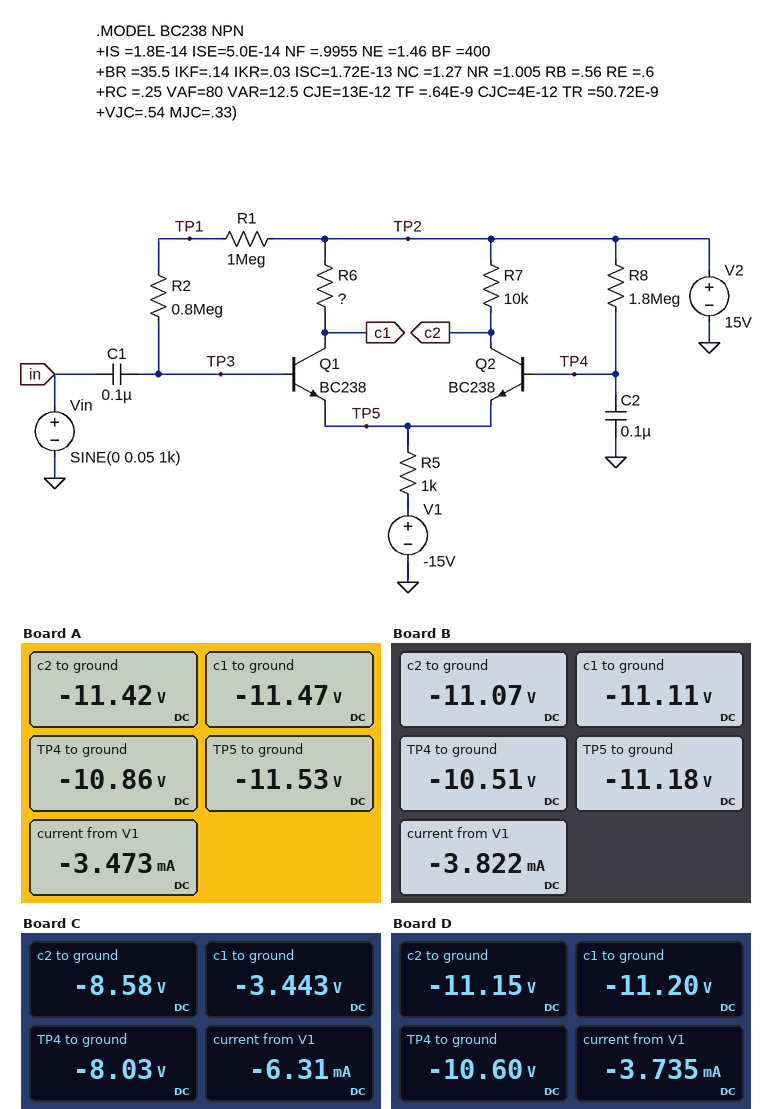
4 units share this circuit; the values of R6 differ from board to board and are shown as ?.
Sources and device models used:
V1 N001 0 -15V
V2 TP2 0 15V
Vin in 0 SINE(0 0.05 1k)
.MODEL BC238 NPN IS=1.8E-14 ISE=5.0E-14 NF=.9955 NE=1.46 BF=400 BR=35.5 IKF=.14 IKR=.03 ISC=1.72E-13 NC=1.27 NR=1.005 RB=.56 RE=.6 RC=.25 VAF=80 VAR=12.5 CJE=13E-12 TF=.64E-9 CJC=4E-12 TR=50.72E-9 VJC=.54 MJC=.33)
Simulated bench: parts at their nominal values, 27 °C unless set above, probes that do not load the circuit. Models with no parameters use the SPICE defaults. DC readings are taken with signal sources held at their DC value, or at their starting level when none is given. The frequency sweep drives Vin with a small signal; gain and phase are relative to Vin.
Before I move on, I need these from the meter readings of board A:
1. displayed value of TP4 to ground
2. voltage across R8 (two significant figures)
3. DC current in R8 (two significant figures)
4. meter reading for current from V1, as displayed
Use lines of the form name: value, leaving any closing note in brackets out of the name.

displayed value of TP4 to ground: -10.86 V
voltage across R8: 26 V
DC current in R8: 14 µA
meter reading for current from V1, as displayed: -3.473 mA
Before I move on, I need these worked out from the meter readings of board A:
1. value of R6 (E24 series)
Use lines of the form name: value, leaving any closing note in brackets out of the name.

value of R6: 33 kΩ
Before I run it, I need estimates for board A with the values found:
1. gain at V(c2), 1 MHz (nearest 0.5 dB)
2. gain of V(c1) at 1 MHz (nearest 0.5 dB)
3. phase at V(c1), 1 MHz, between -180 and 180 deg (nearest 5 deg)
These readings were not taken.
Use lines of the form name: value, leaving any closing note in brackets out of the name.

gain at V(c2), 1 MHz: 23.0 dB
gain of V(c1) at 1 MHz: 14.5 dB
phase at V(c1), 1 MHz, between -180 and 180 deg: 155 deg
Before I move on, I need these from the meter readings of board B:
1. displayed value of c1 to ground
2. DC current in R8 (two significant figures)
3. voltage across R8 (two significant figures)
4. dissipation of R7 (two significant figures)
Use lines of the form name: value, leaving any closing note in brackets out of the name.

displayed value of c1 to ground: -11.11 V
DC current in R8: 14 µA
voltage across R8: 26 V
dissipation of R7: 68 mW
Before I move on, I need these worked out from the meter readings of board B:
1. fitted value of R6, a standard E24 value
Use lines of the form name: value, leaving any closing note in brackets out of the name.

fitted value of R6, a standard E24 value: 22 kΩ
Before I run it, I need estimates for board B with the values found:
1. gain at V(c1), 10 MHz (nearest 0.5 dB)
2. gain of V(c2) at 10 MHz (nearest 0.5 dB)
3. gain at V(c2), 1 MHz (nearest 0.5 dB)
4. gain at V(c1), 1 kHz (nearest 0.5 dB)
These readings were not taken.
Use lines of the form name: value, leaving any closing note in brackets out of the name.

gain at V(c1), 10 MHz: 9.0 dB
gain of V(c2) at 10 MHz: 16.0 dB
gain at V(c2), 1 MHz: 25.0 dB
gain at V(c1), 1 kHz: 1.0 dB
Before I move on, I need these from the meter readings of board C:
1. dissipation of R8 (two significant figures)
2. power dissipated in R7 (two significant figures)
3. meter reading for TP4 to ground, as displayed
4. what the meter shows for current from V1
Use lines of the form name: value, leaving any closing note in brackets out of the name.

dissipation of R8: 290 µW
power dissipated in R7: 56 mW
meter reading for TP4 to ground, as displayed: -8.03 V
what the meter shows for current from V1: -6.31 mA
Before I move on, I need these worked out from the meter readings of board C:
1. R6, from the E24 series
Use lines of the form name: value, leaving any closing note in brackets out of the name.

R6, from the E24 series: 4.7 kΩ
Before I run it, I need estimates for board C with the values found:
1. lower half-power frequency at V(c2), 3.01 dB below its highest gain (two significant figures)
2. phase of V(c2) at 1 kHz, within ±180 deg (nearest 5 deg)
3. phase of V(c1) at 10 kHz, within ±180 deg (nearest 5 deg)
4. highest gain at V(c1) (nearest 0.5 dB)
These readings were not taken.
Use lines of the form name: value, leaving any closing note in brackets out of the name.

lower half-power frequency at V(c2), 3.01 dB below its highest gain: 12 kHz
phase of V(c2) at 1 kHz, within ±180 deg: 75 deg
phase of V(c1) at 10 kHz, within ±180 deg: -135 deg
highest gain at V(c1): 46.0 dB
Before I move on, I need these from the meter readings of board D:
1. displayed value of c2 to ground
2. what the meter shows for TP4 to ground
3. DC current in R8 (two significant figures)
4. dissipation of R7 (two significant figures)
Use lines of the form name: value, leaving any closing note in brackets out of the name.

displayed value of c2 to ground: -11.15 V
what the meter shows for TP4 to ground: -10.60 V
DC current in R8: 14 µA
dissipation of R7: 68 mW
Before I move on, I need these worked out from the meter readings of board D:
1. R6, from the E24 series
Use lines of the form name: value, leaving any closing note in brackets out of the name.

R6, from the E24 series: 24 kΩ
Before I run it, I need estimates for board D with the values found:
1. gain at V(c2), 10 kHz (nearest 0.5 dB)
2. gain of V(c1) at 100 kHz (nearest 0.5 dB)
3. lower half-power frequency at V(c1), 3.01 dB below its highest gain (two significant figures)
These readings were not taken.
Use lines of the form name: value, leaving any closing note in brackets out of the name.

gain at V(c2), 10 kHz: 20.0 dB
gain of V(c1) at 100 kHz: 19.0 dB
lower half-power frequency at V(c1), 3.01 dB below its highest gain: 8.6 kHz
